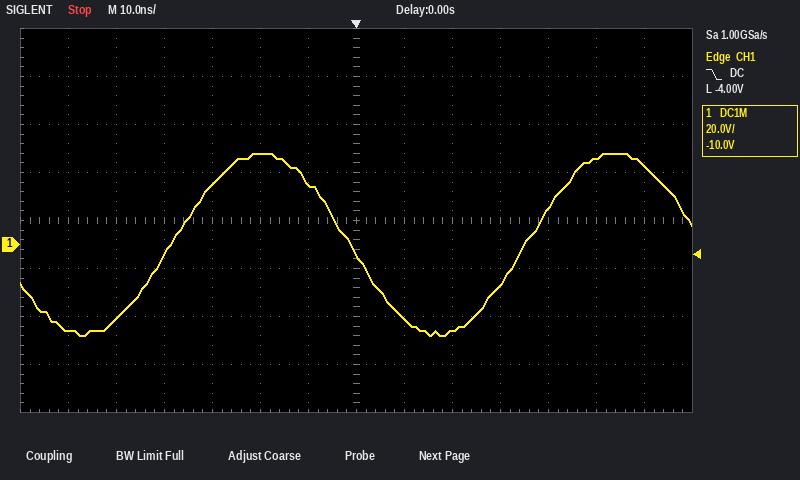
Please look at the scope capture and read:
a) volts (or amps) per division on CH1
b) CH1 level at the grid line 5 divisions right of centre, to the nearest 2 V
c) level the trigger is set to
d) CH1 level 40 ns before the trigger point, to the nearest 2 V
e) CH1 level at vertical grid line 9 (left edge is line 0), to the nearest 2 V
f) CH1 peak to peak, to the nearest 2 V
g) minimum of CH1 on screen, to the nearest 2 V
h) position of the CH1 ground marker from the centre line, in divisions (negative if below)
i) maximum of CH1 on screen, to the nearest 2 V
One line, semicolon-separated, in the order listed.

20 V; 36 V; -4.00 V; -4 V; -36 V; 76 V; -38 V; -0.5 div; 38 V
